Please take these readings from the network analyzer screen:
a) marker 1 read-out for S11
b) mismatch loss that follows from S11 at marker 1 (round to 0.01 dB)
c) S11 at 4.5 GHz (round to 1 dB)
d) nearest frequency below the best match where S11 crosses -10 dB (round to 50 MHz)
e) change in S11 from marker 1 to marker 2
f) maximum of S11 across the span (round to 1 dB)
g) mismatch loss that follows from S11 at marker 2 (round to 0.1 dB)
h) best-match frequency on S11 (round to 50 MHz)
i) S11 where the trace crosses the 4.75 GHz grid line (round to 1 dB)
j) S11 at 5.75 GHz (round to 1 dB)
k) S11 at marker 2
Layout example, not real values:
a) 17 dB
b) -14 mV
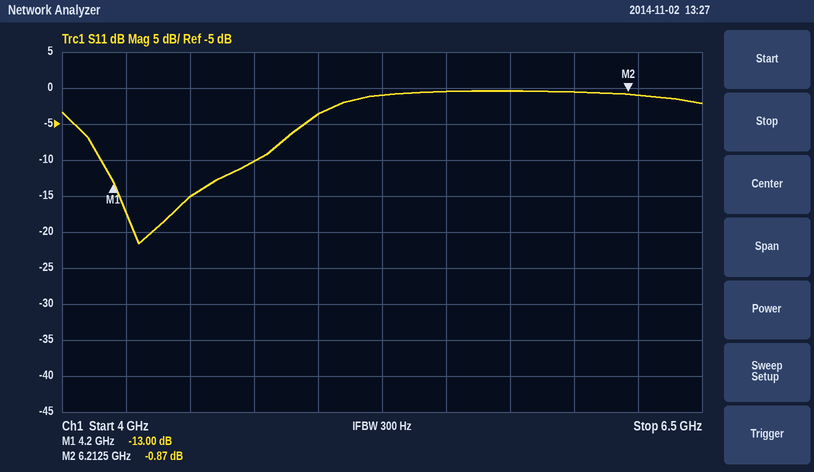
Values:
a) -13.00 dB
b) 0.22 dB
c) -15 dB
d) 4.15 GHz
e) 12.13 dB
f) 0 dB
g) 7.4 dB
h) 4.30 GHz
i) -10 dB
j) 0 dB
k) -0.87 dB
